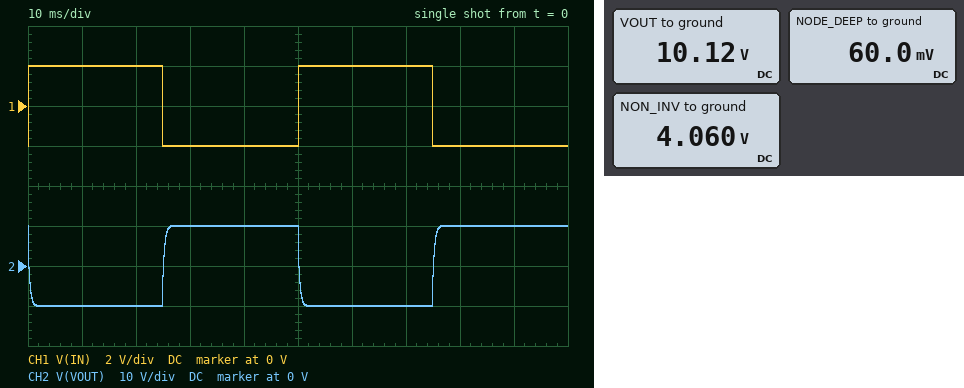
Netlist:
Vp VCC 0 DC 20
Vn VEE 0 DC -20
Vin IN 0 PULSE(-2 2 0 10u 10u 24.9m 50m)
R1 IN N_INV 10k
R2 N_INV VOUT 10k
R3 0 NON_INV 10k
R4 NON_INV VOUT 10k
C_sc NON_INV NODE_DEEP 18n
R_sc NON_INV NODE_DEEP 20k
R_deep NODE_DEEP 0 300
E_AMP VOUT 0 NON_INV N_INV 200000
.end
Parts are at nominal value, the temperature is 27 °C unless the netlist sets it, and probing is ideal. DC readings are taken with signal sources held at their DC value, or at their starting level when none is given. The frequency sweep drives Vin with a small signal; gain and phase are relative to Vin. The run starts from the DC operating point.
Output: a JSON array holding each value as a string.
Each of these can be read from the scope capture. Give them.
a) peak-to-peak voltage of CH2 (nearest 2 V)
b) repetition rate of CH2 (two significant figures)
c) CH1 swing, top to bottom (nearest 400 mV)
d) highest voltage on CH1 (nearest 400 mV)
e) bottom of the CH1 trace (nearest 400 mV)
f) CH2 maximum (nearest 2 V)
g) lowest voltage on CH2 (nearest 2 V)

["20 V", "20 Hz", "4.0 V", "2.0 V", "-2.0 V", "10 V", "-10 V"]
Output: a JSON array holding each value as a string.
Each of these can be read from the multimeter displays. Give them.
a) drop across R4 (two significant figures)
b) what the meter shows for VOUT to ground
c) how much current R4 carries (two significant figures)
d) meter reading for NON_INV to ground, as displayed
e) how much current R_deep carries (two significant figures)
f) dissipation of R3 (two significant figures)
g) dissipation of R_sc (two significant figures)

["6.1 V", "10.12 V", "610 µA", "4.060 V", "200 µA", "1.6 mW", "800 µW"]
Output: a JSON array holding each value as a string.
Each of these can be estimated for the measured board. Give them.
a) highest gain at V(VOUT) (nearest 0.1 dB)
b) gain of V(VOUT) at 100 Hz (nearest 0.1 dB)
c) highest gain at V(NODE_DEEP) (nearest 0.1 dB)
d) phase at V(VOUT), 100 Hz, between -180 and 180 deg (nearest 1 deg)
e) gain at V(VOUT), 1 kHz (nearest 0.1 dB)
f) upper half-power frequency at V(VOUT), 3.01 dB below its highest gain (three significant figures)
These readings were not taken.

["14.1 dB", "13.9 dB", "-30.5 dB", "170 deg", "7.1 dB", "463 Hz"]
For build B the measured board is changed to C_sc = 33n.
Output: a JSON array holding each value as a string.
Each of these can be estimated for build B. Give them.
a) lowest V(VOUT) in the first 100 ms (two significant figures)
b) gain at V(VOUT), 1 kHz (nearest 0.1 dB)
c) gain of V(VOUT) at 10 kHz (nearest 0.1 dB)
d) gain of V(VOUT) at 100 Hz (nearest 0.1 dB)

["-10 V", "3.9 dB", "0.6 dB", "13.4 dB"]
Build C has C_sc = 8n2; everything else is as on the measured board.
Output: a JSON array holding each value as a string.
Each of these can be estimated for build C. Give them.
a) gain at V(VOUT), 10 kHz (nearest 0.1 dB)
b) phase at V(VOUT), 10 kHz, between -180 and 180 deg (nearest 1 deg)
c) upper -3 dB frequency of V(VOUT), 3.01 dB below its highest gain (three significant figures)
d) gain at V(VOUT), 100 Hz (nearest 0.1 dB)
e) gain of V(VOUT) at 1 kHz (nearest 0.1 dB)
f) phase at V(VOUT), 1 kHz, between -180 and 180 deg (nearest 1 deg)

["1.3 dB", "161 deg", "1.02 kHz", "14.0 dB", "11.1 dB", "146 deg"]
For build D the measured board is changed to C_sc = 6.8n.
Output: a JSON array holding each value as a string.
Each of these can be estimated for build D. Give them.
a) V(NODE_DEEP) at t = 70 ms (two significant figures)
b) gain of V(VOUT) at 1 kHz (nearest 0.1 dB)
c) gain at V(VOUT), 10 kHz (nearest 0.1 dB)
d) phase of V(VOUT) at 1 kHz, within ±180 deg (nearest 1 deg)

["-60 mV", "11.8 dB", "1.6 dB", "150 deg"]
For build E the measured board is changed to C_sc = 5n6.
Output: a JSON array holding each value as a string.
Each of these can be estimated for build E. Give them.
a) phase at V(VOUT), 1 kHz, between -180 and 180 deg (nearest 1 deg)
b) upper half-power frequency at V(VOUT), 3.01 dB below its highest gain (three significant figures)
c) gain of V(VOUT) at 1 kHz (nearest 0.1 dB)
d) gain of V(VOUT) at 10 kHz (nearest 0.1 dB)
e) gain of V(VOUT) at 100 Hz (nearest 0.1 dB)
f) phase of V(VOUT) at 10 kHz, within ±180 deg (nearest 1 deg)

["153 deg", "1.49 kHz", "12.4 dB", "2.1 dB", "14.1 dB", "154 deg"]
